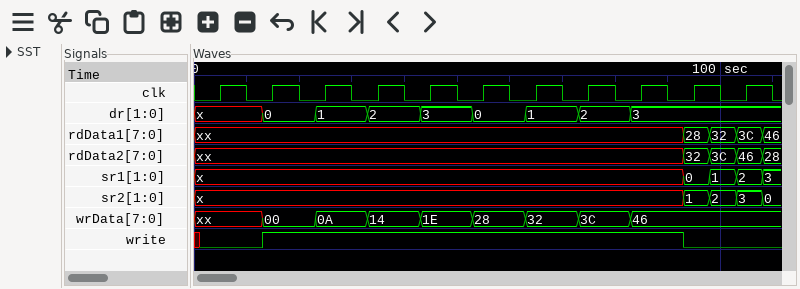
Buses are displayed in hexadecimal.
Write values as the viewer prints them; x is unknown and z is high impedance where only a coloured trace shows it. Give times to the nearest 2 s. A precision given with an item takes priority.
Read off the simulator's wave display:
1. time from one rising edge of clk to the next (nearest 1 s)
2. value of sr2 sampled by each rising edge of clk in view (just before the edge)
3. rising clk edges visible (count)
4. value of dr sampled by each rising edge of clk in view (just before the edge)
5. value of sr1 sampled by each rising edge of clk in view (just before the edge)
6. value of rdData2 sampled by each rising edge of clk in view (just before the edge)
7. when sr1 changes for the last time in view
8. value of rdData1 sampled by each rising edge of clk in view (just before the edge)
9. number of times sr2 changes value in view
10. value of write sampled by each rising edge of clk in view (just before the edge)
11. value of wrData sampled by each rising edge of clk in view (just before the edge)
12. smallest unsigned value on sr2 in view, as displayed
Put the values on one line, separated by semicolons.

10 s; x, x, x, x, x, x, x, x, x, 1, 3; 11; x, 0, 1, 2, 3, 0, 1, 2, 3, 3, 3; x, x, x, x, x, x, x, x, x, 0, 2; xx, xx, xx, xx, xx, xx, xx, xx, xx, 32, 46; 108 s; xx, xx, xx, xx, xx, xx, xx, xx, xx, 28, 3C; 4; 0 1 1 1 1 1 1 1 1 0 0; xx, 00, 0A, 14, 1E, 28, 32, 3C, 46, 46, 46; 0
